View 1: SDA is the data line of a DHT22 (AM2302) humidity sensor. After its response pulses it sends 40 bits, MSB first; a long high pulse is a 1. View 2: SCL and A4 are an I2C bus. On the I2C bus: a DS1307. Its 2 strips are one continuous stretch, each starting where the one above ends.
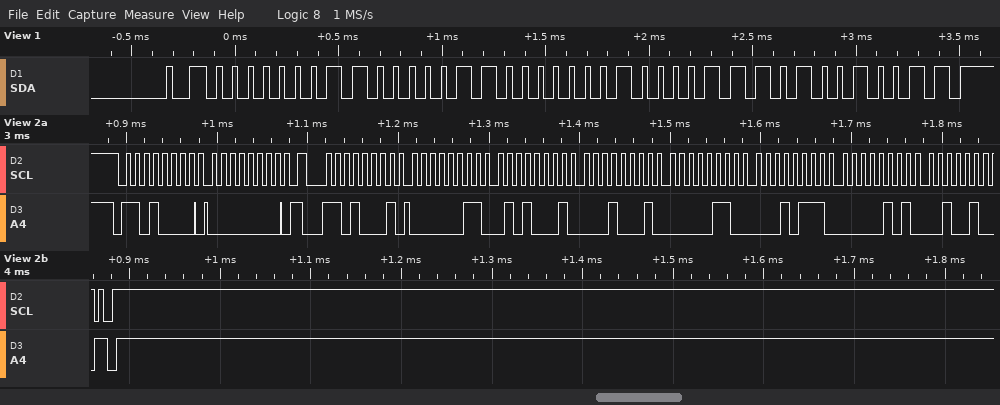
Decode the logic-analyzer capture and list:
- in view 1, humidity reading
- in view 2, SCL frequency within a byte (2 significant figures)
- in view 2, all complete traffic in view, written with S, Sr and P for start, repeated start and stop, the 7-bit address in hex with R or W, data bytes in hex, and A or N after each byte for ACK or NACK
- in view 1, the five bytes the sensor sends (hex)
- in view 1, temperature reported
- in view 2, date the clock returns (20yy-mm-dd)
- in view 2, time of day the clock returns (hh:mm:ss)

38.7 %
100 kHz
S 68W A 00 A Sr 68R A 03 A 51 A 11 A 06 A 17 A 05 A 24 N P
01 83 01 0E 93
27.0 °C
2024-05-17
11:51:03
